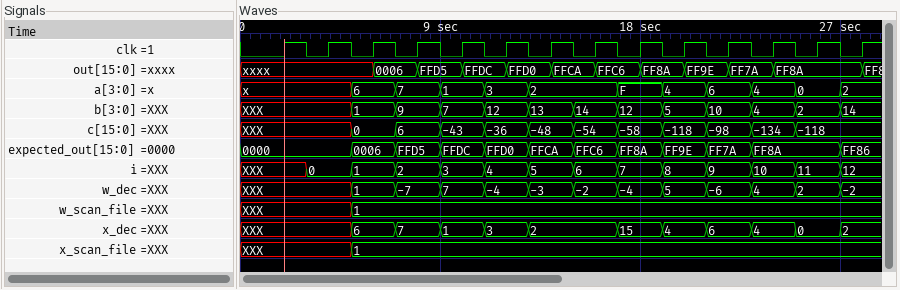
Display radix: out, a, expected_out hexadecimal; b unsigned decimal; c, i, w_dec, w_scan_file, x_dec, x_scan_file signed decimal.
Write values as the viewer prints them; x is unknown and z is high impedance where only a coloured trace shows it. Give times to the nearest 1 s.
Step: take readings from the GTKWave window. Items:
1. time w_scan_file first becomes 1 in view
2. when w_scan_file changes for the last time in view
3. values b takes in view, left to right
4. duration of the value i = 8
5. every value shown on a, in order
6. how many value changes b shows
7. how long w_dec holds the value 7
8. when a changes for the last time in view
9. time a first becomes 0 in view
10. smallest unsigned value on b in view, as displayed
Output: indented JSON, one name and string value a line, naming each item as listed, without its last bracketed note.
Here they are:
{
  "time w_scan_file first becomes 1 in view": "5 s",
  "when w_scan_file changes for the last time in view": "5 s",
  "values b takes in view, left to right": "XXX, 1, 9, 7, 12, 13, 14, 12, 5, 10, 4, 2, 14",
  "duration of the value i = 8": "2 s",
  "every value shown on a, in order": "x, 6, 7, 1, 3, 2, F, 4, 6, 4, 0, 2",
  "how many value changes b shows": "12",
  "how long w_dec holds the value 7": "2 s",
  "when a changes for the last time in view": "27 s",
  "time a first becomes 0 in view": "25 s",
  "smallest unsigned value on b in view, as displayed": "1"
}
